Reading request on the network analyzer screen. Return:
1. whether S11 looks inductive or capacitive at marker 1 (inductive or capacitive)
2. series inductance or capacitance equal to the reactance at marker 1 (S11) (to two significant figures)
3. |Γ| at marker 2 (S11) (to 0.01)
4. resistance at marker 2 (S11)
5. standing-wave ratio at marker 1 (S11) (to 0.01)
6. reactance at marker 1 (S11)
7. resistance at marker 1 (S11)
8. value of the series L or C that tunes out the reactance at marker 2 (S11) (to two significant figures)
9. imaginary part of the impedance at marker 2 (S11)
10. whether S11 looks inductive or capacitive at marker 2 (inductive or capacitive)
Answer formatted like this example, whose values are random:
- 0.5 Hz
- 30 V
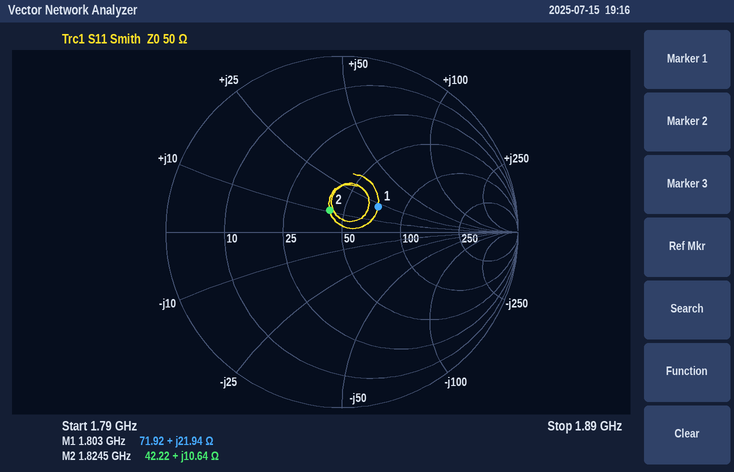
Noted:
- inductive
- 1.9 nH
- 0.14
- 42.22 Ω
- 1.67
- +21.94 Ω
- 71.92 Ω
- 8.2 pF
- +10.64 Ω
- inductive
